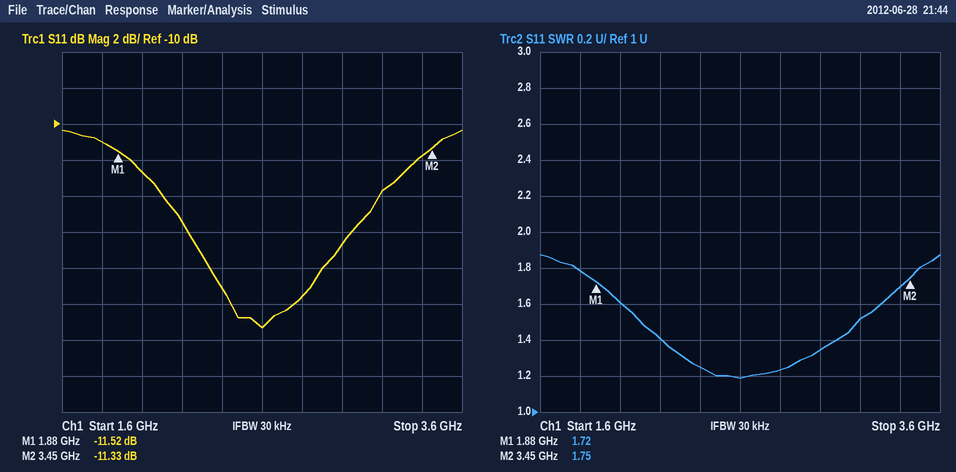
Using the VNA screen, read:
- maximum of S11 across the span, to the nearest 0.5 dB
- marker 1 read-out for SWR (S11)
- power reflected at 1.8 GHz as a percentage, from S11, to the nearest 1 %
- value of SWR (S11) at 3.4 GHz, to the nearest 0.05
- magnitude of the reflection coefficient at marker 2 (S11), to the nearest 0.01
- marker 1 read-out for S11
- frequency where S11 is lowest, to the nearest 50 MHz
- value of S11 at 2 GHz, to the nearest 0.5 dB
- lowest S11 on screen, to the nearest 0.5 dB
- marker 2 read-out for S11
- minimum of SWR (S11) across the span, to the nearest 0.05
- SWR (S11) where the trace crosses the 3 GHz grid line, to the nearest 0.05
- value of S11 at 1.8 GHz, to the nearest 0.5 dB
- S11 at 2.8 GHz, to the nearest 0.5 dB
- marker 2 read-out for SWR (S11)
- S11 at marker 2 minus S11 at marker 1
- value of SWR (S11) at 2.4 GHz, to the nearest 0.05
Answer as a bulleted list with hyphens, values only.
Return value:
- -10.5 dB
- 1.72
- 8 %
- 1.70
- 0.27
- -11.52 dB
- 2.60 GHz
- -12.5 dB
- -21.5 dB
- -11.33 dB
- 1.20
- 1.35
- -11.0 dB
- -19.5 dB
- 1.75
- 0.19 dB
- 1.25
